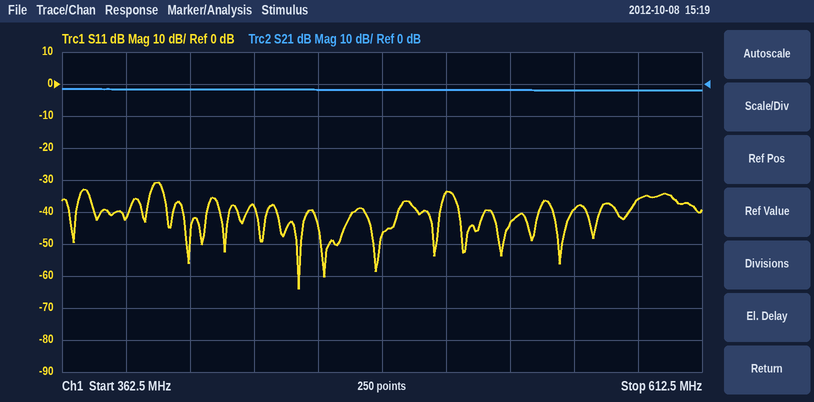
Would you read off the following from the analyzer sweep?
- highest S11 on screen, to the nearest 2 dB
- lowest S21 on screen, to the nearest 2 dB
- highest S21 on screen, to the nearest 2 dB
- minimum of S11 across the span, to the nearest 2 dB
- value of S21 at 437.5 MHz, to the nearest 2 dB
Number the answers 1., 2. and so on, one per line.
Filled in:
1. -30 dB
2. -2 dB
3. -2 dB
4. -64 dB
5. -2 dB
